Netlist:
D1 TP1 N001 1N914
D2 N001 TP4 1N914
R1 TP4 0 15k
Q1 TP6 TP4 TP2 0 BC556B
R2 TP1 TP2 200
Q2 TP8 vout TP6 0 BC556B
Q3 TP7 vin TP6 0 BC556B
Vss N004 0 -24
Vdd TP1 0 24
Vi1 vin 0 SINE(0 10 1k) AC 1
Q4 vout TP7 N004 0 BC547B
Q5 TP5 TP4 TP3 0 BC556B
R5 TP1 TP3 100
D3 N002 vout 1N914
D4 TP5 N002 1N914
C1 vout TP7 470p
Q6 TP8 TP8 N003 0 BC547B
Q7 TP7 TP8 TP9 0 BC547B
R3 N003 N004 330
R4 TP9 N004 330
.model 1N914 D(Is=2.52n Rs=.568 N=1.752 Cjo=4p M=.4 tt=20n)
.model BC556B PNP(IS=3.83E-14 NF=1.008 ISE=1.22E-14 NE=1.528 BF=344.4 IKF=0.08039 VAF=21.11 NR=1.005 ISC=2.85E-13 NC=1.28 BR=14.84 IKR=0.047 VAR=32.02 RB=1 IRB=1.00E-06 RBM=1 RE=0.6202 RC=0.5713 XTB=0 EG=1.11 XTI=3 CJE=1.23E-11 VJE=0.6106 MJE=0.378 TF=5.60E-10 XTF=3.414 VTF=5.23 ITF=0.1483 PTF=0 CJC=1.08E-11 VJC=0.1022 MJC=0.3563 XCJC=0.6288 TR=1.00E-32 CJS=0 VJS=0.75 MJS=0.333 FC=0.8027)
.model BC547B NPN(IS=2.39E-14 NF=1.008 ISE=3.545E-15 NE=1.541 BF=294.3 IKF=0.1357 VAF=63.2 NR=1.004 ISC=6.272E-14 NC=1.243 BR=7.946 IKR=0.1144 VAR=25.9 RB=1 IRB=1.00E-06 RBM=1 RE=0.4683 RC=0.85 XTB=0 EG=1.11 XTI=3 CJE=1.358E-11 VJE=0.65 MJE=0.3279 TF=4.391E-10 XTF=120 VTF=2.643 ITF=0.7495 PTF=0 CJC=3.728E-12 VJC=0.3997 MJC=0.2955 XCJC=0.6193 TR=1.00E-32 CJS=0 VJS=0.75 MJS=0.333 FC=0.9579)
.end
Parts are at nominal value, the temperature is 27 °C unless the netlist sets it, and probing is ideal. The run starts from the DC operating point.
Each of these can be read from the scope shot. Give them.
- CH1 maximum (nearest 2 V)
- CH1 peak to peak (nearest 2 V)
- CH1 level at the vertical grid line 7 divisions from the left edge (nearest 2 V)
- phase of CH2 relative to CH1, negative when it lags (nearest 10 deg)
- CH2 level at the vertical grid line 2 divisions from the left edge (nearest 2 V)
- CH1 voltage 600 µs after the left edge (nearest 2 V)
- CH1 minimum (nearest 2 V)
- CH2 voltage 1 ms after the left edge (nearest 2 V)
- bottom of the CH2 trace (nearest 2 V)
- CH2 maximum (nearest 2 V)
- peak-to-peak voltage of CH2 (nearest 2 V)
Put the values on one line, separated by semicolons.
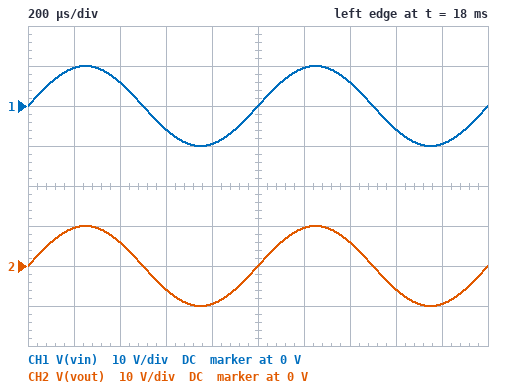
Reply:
10 V; 20 V; 6 V; 0 deg; 6 V; -6 V; -10 V; 0 V; -10 V; 10 V; 20 V
